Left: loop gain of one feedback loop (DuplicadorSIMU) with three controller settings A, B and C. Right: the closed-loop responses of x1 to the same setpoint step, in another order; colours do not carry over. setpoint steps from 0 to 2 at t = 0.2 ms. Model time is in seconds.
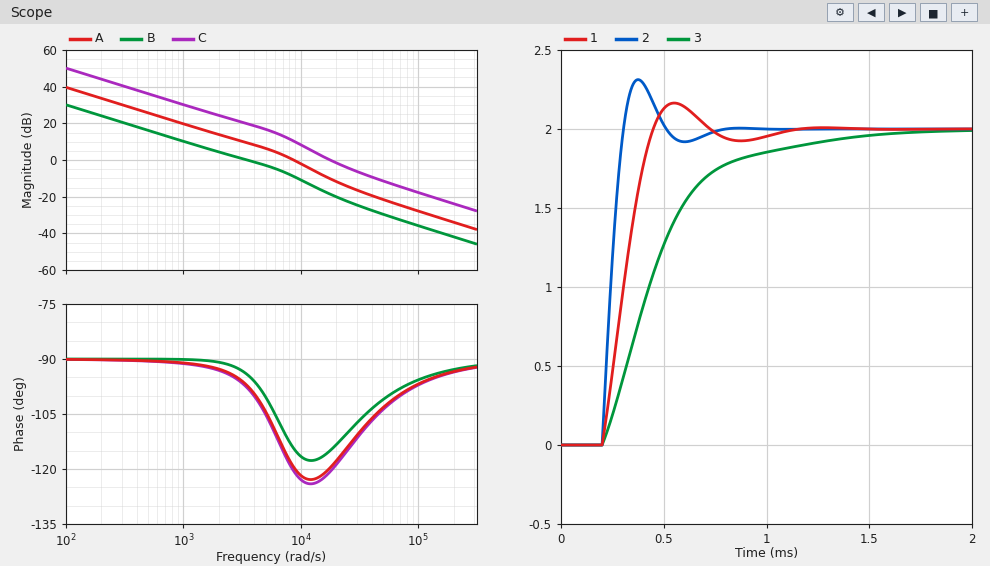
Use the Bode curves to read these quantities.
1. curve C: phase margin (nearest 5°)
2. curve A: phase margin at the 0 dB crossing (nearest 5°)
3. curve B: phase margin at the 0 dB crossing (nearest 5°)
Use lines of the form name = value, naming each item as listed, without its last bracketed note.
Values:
curve C: phase margin = 60°
curve A: phase margin at the 0 dB crossing = 60°
curve B: phase margin at the 0 dB crossing = 85°
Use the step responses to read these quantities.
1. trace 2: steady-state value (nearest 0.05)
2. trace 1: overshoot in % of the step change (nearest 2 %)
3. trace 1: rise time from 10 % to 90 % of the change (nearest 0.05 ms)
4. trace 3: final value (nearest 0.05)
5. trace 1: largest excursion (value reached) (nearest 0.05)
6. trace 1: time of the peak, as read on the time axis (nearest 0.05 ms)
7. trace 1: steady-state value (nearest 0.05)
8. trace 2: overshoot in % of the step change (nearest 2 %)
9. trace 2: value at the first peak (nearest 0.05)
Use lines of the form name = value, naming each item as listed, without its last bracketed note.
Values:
trace 2: steady-state value = 2.00
trace 1: overshoot in % of the step change = 8 %
trace 1: rise time from 10 % to 90 % of the change = 0.20 ms
trace 3: final value = 2.00
trace 1: largest excursion (value reached) = 2.15
trace 1: time of the peak, as read on the time axis = 0.55 ms
trace 1: steady-state value = 2.00
trace 2: overshoot in % of the step change = 16 %
trace 2: value at the first peak = 2.30
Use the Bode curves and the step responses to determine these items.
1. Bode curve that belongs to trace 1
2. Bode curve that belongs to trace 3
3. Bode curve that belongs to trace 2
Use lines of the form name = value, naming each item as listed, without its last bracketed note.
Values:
Bode curve that belongs to trace 1 = A
Bode curve that belongs to trace 3 = B
Bode curve that belongs to trace 2 = C
